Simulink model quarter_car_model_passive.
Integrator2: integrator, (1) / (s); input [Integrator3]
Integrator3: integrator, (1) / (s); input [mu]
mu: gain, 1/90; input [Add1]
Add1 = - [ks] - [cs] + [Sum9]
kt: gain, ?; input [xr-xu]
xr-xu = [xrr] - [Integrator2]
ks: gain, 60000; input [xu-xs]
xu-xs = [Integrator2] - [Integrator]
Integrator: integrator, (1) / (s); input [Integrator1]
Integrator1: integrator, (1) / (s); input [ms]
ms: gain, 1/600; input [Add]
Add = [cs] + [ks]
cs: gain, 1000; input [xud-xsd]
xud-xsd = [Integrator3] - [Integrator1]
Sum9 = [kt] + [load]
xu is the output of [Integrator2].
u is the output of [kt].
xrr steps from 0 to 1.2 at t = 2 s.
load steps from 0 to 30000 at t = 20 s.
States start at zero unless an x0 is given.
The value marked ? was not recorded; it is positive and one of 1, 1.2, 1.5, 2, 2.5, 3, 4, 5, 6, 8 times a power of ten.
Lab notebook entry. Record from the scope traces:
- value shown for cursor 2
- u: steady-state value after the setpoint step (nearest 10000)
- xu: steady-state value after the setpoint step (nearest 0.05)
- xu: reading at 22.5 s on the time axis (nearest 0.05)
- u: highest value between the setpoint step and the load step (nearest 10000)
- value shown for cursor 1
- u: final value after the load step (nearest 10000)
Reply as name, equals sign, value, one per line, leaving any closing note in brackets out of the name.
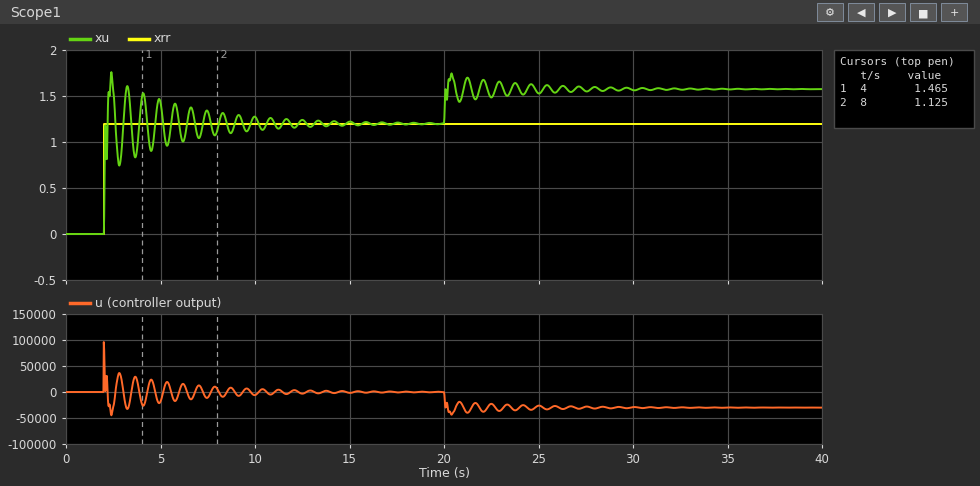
value shown for cursor 2 = 1.125
u: steady-state value after the setpoint step = 0
xu: steady-state value after the setpoint step = 1.20
xu: reading at 22.5 s on the time axis = 1.50
u: highest value between the setpoint step and the load step = 100000
value shown for cursor 1 = 1.465
u: final value after the load step = -30000
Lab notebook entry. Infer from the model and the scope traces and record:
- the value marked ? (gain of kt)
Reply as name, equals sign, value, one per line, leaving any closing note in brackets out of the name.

the value marked ? = 80000
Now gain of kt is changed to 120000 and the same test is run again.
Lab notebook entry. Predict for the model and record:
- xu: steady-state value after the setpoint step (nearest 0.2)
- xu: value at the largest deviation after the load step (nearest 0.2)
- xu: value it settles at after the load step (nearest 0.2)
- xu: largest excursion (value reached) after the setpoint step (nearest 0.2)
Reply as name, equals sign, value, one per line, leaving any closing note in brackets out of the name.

xu: steady-state value after the setpoint step = 1.2
xu: value at the largest deviation after the load step = 1.6
xu: value it settles at after the load step = 1.4
xu: largest excursion (value reached) after the setpoint step = 1.6
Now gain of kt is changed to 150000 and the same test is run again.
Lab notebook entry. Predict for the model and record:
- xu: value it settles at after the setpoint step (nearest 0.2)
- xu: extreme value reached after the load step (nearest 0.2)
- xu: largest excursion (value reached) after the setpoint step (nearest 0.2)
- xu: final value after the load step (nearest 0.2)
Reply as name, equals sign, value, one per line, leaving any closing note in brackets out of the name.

xu: value it settles at after the setpoint step = 1.2
xu: extreme value reached after the load step = 1.4
xu: largest excursion (value reached) after the setpoint step = 1.6
xu: final value after the load step = 1.4
